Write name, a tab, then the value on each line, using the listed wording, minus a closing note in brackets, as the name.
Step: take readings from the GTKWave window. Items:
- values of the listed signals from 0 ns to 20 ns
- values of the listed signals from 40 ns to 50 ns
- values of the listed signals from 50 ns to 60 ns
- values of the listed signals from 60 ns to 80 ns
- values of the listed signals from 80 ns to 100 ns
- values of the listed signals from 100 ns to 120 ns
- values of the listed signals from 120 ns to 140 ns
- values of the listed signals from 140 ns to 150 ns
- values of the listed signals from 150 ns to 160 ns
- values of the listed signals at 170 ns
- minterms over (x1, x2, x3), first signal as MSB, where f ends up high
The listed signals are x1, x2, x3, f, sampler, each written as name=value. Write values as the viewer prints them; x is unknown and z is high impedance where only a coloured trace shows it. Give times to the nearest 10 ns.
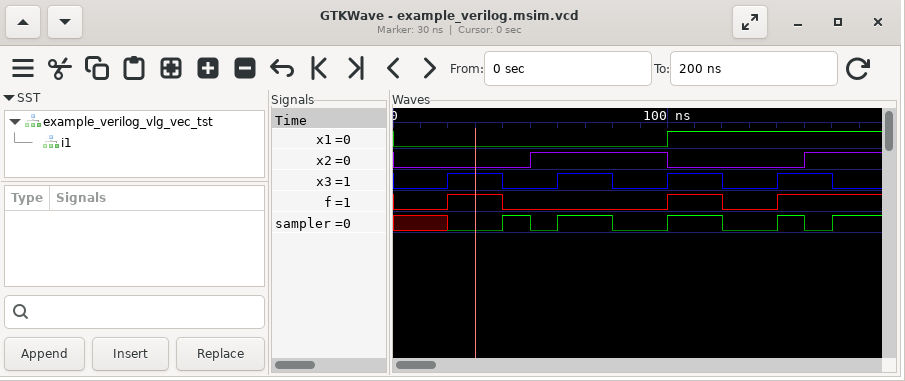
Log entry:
values of the listed signals from 0 ns to 20 ns	x1=0, x2=0, x3=0, f=0, sampler=x
values of the listed signals from 40 ns to 50 ns	x1=0, x2=0, x3=0, f=0, sampler=1
values of the listed signals from 50 ns to 60 ns	x1=0, x2=1, x3=0, f=0, sampler=0
values of the listed signals from 60 ns to 80 ns	x1=0, x2=1, x3=1, f=0, sampler=1
values of the listed signals from 80 ns to 100 ns	x1=0, x2=1, x3=0, f=0, sampler=0
values of the listed signals from 100 ns to 120 ns	x1=1, x2=0, x3=1, f=1, sampler=1
values of the listed signals from 120 ns to 140 ns	x1=1, x2=0, x3=0, f=0, sampler=0
values of the listed signals from 140 ns to 150 ns	x1=1, x2=0, x3=1, f=1, sampler=1
values of the listed signals from 150 ns to 160 ns	x1=1, x2=1, x3=1, f=1, sampler=0
values of the listed signals at 170 ns	x1=1, x2=1, x3=0, f=1, sampler=1
minterms over (x1, x2, x3), first signal as MSB, where f ends up high	1, 5, 6, 7
